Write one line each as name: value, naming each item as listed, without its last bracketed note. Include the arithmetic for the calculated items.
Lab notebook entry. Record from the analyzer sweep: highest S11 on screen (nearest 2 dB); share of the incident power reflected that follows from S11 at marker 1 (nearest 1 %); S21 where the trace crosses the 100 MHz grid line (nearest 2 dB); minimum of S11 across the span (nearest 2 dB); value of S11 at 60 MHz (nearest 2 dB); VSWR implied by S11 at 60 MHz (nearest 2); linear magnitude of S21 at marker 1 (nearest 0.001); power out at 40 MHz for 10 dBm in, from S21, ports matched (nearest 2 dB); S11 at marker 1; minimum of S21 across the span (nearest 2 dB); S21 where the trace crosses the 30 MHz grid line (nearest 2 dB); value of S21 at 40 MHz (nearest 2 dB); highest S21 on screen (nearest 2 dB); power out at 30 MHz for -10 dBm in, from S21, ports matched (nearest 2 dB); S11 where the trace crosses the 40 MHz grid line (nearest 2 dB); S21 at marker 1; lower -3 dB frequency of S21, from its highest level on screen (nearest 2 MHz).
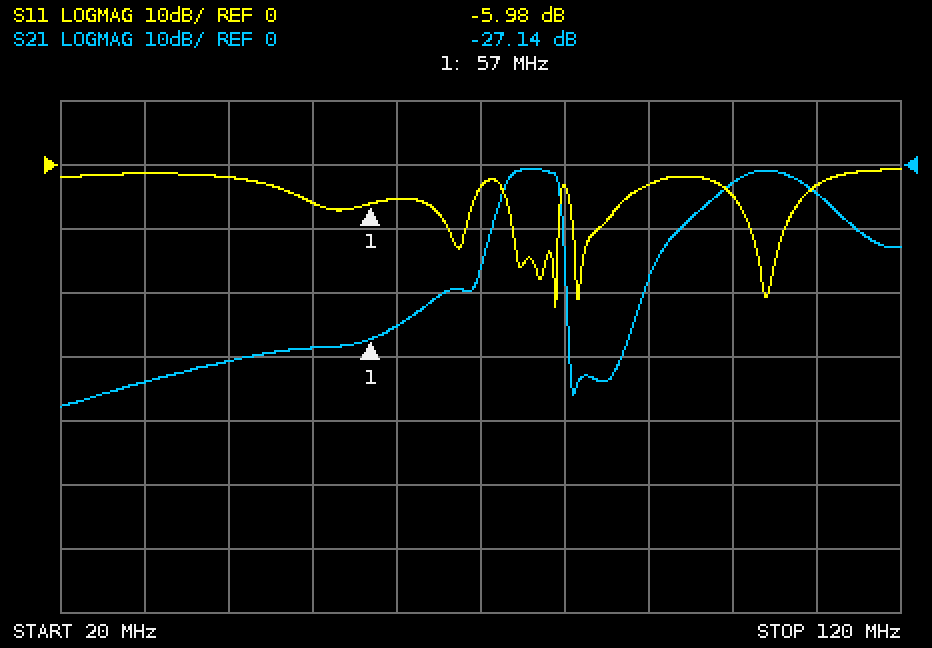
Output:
highest S11 on screen: 0 dB
share of the incident power reflected that follows from S11 at marker 1: 10^(-5.98/10) ≈ 25 %
S21 where the trace crosses the 100 MHz grid line: -2 dB
minimum of S11 across the span: -22 dB
value of S11 at 60 MHz: -6 dB
VSWR implied by S11 at 60 MHz: |Γ| = 10^(-6/20) = 0.5012; VSWR = (1 + 0.5012)/(1 − 0.5012) ≈ 3.01, so 4 to the nearest 2
linear magnitude of S21 at marker 1: 10^(-27.14/20) ≈ 0.044
power out at 40 MHz for 10 dBm in, from S21, ports matched: 10 dBm + (-30 dB) = -20 dBm
S11 at marker 1: -5.98 dB
minimum of S21 across the span: -38 dB
S21 where the trace crosses the 30 MHz grid line: -34 dB
value of S21 at 40 MHz: -30 dB
highest S21 on screen: 0 dB
power out at 30 MHz for -10 dBm in, from S21, ports matched: -10 dBm + (-34 dB) = -44 dBm
S11 where the trace crosses the 40 MHz grid line: -2 dB
S21 at marker 1: -27.14 dB
lower -3 dB frequency of S21, from its highest level on screen: 72 MHz
